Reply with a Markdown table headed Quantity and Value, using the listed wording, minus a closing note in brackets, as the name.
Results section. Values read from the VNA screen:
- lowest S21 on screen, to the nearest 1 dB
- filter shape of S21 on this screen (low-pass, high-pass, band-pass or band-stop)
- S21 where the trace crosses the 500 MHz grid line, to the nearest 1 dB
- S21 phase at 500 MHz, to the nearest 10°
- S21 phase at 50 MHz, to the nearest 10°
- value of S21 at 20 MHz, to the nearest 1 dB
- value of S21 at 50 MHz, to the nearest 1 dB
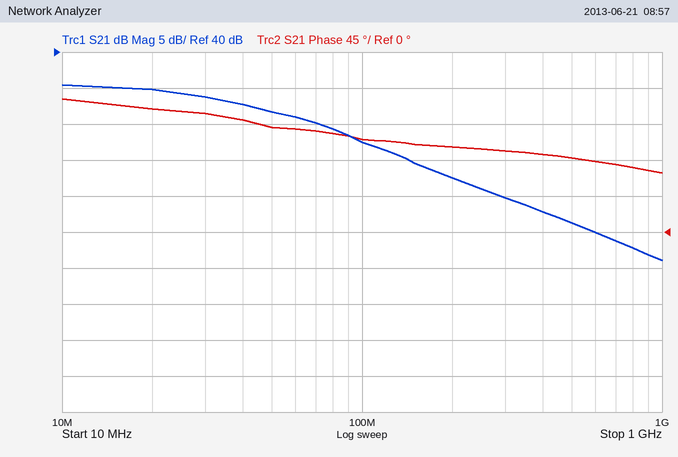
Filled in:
| Quantity | Value |
|---|---|
| lowest S21 on screen, to the nearest 1 dB | 11 dB |
| filter shape of S21 on this screen | low-pass |
| S21 where the trace crosses the 500 MHz grid line, to the nearest 1 dB | 16 dB |
| S21 phase at 500 MHz, to the nearest 10° | 90° |
| S21 phase at 50 MHz, to the nearest 10° | 130° |
| value of S21 at 20 MHz, to the nearest 1 dB | 35 dB |
| value of S21 at 50 MHz, to the nearest 1 dB | 32 dB |
